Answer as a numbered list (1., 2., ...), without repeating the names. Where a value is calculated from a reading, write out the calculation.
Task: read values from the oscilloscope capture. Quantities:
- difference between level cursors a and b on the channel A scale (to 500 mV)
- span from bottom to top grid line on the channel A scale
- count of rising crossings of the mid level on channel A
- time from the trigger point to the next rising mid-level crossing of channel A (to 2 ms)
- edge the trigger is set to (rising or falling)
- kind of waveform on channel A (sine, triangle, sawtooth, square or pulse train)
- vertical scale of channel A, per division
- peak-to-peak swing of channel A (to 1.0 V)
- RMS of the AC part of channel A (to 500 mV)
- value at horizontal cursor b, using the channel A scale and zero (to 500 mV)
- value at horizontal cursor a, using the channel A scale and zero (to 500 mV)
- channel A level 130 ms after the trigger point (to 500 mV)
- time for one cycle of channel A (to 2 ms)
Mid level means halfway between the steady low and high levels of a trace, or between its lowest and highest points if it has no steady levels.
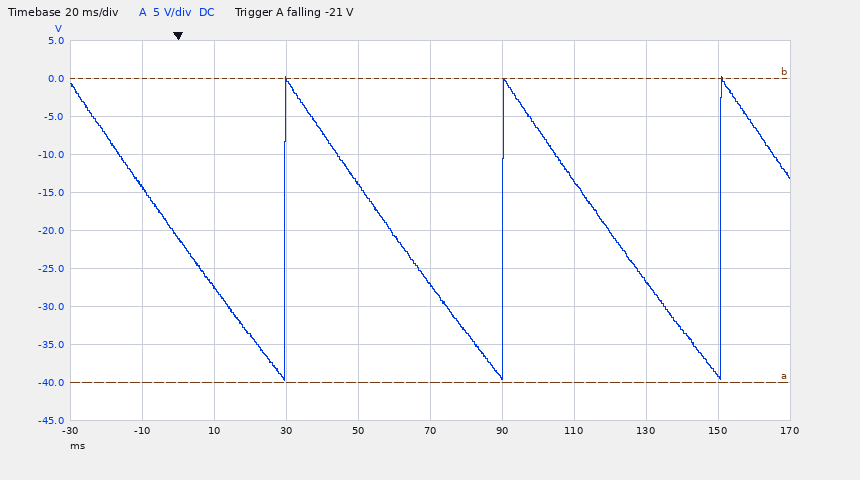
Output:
1. 40.0 V
2. 50 V
3. 3
4. 30 ms
5. falling
6. sawtooth
7. 5 V
8. 40.0 V
9. 40.0 V / (2√3) ≈ 11.5 V
10. 0.0 V
11. -40.0 V
12. -26.5 V
13. 60 ms
